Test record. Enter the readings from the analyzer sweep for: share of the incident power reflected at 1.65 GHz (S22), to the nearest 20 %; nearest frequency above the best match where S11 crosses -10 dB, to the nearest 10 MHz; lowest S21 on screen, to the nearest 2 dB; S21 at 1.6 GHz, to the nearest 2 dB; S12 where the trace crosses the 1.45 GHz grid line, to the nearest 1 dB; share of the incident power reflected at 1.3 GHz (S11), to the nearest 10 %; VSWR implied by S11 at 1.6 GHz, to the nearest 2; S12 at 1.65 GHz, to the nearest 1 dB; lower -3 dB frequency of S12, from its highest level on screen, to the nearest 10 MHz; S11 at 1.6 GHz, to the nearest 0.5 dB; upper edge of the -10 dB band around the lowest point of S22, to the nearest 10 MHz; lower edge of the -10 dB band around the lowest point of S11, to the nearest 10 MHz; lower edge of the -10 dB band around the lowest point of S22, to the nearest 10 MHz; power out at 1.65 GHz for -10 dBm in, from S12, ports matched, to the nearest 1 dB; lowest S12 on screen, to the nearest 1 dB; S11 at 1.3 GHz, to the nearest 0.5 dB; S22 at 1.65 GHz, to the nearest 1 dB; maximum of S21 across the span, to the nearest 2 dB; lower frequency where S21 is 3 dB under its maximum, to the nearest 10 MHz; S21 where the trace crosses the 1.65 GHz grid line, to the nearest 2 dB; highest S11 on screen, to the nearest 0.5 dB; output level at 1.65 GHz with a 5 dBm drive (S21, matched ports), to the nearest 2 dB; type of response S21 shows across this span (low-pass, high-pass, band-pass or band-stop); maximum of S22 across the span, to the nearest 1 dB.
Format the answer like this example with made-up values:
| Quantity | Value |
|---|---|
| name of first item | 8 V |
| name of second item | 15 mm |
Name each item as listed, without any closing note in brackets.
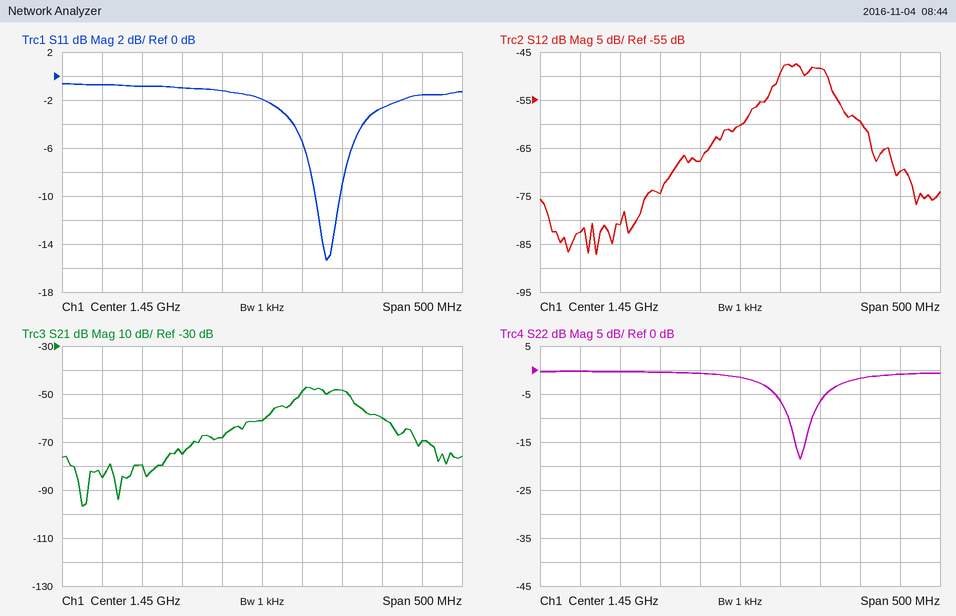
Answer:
| Quantity | Value |
|---|---|
| share of the incident power reflected at 1.65 GHz (S22), to the nearest 20 % | 80 % |
| nearest frequency above the best match where S11 crosses -10 dB, to the nearest 10 MHz | 1.55 GHz |
| lowest S21 on screen, to the nearest 2 dB | -96 dB |
| S21 at 1.6 GHz, to the nearest 2 dB | -60 dB |
| S12 where the trace crosses the 1.45 GHz grid line, to the nearest 1 dB | -60 dB |
| share of the incident power reflected at 1.3 GHz (S11), to the nearest 10 % | 80 % |
| VSWR implied by S11 at 1.6 GHz, to the nearest 2 | 6 |
| S12 at 1.65 GHz, to the nearest 1 dB | -70 dB |
| lower -3 dB frequency of S12, from its highest level on screen, to the nearest 10 MHz | 1.50 GHz |
| S11 at 1.6 GHz, to the nearest 0.5 dB | -2.5 dB |
| upper edge of the -10 dB band around the lowest point of S22, to the nearest 10 MHz | 1.54 GHz |
| lower edge of the -10 dB band around the lowest point of S11, to the nearest 10 MHz | 1.52 GHz |
| lower edge of the -10 dB band around the lowest point of S22, to the nearest 10 MHz | 1.51 GHz |
| power out at 1.65 GHz for -10 dBm in, from S12, ports matched, to the nearest 1 dB | -80 dBm |
| lowest S12 on screen, to the nearest 1 dB | -87 dB |
| S11 at 1.3 GHz, to the nearest 0.5 dB | -1.0 dB |
| S22 at 1.65 GHz, to the nearest 1 dB | -1 dB |
| maximum of S21 across the span, to the nearest 2 dB | -48 dB |
| lower frequency where S21 is 3 dB under its maximum, to the nearest 10 MHz | 1.50 GHz |
| S21 where the trace crosses the 1.65 GHz grid line, to the nearest 2 dB | -70 dB |
| highest S11 on screen, to the nearest 0.5 dB | -0.5 dB |
| output level at 1.65 GHz with a 5 dBm drive (S21, matched ports), to the nearest 2 dB | -64 dBm |
| type of response S21 shows across this span | band-pass |
| maximum of S22 across the span, to the nearest 1 dB | 0 dB |
